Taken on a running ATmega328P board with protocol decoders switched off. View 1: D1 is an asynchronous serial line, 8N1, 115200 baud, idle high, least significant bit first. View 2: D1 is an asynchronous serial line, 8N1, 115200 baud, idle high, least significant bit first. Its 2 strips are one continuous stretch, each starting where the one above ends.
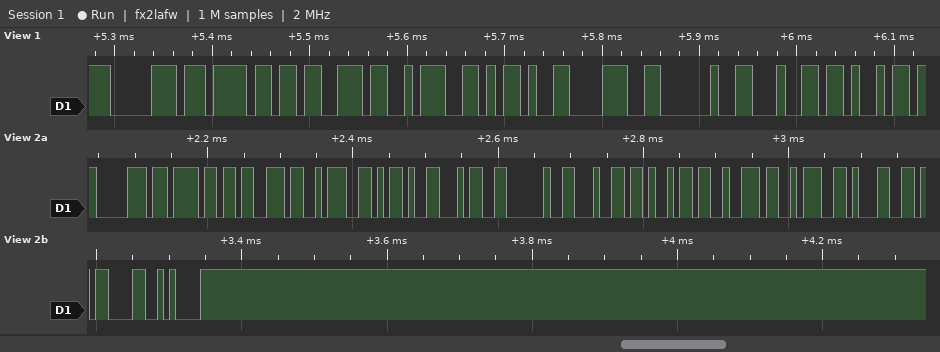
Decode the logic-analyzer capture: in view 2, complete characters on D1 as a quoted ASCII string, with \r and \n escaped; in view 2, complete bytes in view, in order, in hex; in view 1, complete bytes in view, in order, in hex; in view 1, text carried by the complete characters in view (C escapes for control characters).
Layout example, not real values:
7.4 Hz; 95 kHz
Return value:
"pos:-4 dir:1\r\n"; 70 6F 73 3A 2D 34 20 64 69 72 3A 31 0D 0A; 70 6F 73 3A 2D 38 20 64 69; "pos:-8 di"
